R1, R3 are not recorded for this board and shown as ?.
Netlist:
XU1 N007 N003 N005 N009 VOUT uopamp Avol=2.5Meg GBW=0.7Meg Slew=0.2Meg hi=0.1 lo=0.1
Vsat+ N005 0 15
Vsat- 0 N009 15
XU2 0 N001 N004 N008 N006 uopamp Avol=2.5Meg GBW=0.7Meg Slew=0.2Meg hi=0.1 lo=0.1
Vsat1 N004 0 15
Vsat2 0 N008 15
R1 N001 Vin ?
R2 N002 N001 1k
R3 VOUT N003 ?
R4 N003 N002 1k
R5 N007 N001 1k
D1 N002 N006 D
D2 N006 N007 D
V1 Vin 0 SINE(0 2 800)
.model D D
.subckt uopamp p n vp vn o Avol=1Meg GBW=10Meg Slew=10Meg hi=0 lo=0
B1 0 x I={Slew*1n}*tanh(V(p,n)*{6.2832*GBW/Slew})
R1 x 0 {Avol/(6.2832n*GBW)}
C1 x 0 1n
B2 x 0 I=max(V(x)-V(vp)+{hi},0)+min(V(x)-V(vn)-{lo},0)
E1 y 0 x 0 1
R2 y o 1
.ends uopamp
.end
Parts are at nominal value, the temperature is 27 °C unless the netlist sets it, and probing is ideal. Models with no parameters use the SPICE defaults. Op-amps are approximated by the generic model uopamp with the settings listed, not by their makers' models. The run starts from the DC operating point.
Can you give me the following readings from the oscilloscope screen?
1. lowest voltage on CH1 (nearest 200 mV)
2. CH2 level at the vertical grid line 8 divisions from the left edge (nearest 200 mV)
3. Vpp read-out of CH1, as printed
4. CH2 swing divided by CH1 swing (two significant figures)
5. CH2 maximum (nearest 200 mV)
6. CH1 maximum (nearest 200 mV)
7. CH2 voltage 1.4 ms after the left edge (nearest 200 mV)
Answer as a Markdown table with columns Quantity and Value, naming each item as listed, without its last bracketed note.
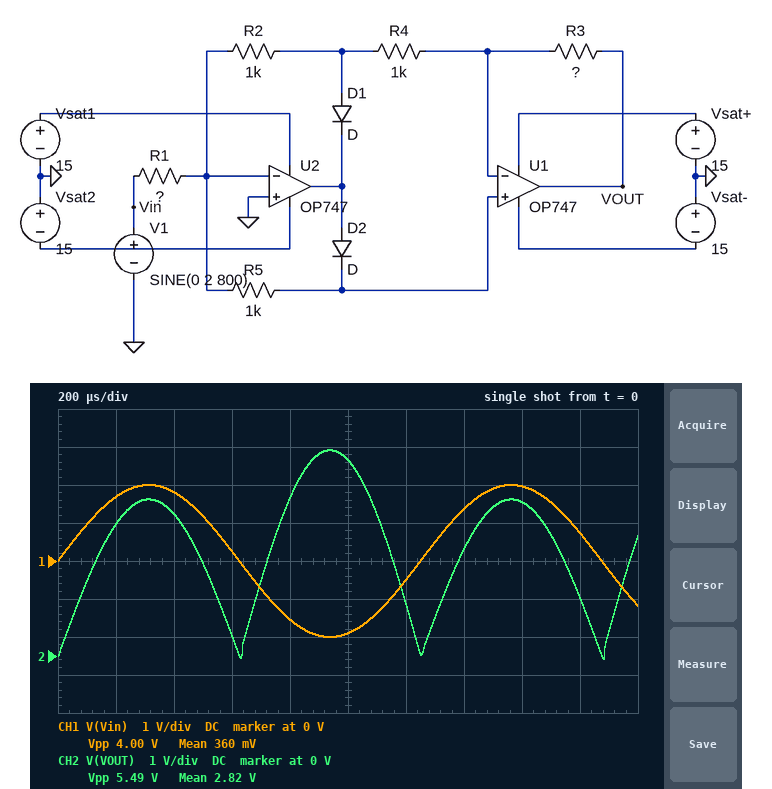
| Quantity | Value |
|---|---|
| lowest voltage on CH1 | -2.0 V |
| CH2 level at the vertical grid line 8 divisions from the left edge | 4.0 V |
| Vpp read-out of CH1, as printed | 4.00 V |
| CH2 swing divided by CH1 swing | 1.4 |
| CH2 maximum | 5.4 V |
| CH1 maximum | 2.0 V |
| CH2 voltage 1.4 ms after the left edge | 2.8 V |
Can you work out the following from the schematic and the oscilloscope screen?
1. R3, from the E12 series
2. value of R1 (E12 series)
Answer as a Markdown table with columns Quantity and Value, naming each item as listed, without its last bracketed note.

| Quantity | Value |
|---|---|
| R3, from the E12 series | 680 Ω |
| value of R1 | 330 Ω |
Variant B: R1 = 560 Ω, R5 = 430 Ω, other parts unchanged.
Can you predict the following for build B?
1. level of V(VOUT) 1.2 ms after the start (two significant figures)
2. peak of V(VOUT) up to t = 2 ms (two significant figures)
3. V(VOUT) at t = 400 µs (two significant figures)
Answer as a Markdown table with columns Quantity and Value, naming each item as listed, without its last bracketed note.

| Quantity | Value |
|---|---|
| level of V(VOUT) 1.2 ms after the start | 430 mV |
| peak of V(VOUT) up to t = 2 ms | 2.4 V |
| V(VOUT) at t = 400 µs | 2.2 V |
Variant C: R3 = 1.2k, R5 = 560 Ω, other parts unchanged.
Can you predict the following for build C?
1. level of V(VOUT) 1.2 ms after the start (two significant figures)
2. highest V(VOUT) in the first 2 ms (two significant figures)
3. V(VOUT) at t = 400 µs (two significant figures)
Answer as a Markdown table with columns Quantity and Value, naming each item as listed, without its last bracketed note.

| Quantity | Value |
|---|---|
| level of V(VOUT) 1.2 ms after the start | 1.1 V |
| highest V(VOUT) in the first 2 ms | 7.3 V |
| V(VOUT) at t = 400 µs | 6.6 V |
